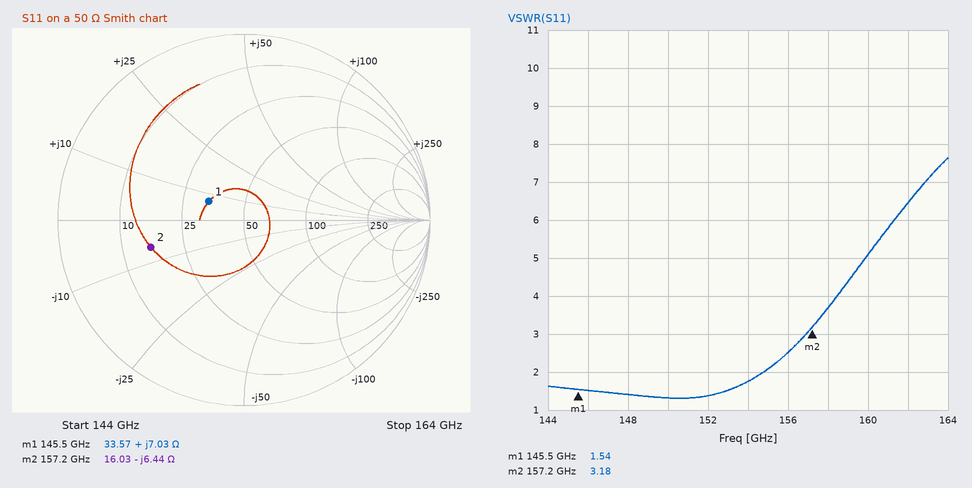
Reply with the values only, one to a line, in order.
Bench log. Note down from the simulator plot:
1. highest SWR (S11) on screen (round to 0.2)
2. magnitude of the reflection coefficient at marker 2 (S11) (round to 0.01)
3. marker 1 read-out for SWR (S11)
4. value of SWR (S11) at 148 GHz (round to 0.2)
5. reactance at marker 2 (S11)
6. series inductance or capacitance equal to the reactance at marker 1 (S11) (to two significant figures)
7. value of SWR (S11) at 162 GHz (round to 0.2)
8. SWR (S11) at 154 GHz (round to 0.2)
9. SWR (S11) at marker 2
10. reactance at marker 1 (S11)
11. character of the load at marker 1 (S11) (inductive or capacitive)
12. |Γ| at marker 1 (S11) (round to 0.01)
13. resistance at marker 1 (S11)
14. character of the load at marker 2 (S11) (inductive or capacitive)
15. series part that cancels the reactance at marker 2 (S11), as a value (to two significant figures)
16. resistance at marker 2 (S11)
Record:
7.6
0.52
1.54
1.4
-6.44 Ω
7.7 pH
6.4
1.8
3.18
+7.03 Ω
inductive
0.21
33.57 Ω
capacitive
6.5 pH
16.03 Ω
